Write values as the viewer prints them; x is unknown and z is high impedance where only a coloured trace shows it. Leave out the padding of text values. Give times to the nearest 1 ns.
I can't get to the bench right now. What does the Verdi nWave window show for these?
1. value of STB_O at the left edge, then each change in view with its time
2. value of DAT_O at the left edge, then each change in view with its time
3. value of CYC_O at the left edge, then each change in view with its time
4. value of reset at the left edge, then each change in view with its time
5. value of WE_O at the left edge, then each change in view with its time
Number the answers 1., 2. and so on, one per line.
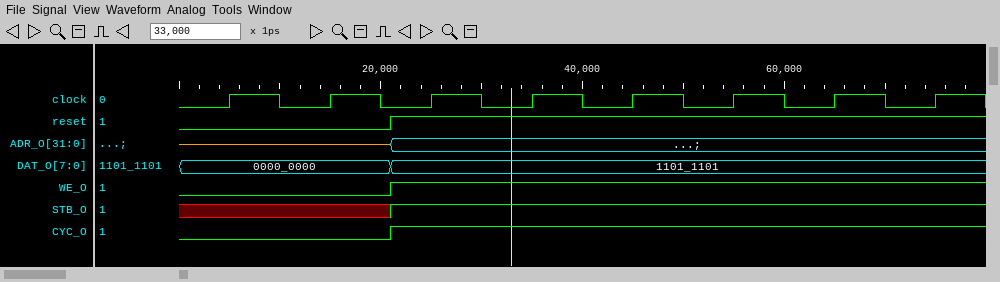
1. x, 1 at 21 ns
2. 0000_0000, 1101_1101 at 21 ns
3. 0, 1 at 21 ns
4. 0, 1 at 21 ns
5. 0, 1 at 21 ns
